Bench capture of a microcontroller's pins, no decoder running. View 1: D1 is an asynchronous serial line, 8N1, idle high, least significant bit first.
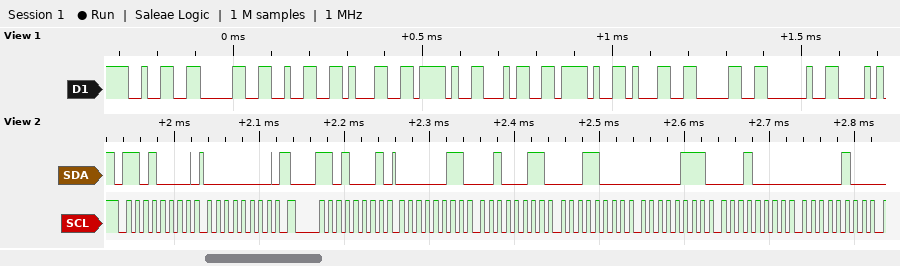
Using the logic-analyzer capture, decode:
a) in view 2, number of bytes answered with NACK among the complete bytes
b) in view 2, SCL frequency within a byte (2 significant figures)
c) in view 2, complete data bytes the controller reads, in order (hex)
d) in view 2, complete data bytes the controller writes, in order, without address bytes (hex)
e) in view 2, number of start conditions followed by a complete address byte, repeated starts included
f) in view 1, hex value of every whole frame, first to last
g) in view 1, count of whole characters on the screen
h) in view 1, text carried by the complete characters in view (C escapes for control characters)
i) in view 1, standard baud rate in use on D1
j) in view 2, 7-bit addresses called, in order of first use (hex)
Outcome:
0
100 kHz
03 23 18 07 10 04
00
2
32 30 32 31 2F 34 2F 31 30 20
10
"2021/4/10 "
57600 baud
0x68
